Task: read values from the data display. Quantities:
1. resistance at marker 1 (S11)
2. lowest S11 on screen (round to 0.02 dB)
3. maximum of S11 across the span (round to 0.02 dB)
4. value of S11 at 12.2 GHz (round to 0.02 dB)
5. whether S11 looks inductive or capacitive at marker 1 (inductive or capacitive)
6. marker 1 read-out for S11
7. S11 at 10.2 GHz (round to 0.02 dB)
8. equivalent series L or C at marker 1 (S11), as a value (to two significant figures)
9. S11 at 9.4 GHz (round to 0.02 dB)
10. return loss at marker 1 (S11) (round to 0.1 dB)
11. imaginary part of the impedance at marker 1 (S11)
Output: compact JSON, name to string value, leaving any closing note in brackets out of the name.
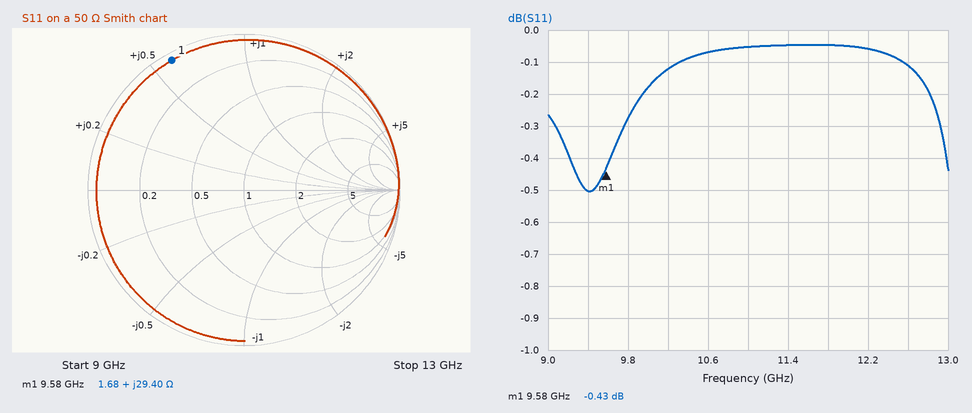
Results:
{"resistance at marker 1": "1.68 Ω", "lowest S11 on screen": "-0.50 dB", "maximum of S11 across the span": "-0.04 dB", "value of S11 at 12.2 GHz": "-0.06 dB", "whether S11 looks inductive or capacitive at marker 1": "inductive", "marker 1 read-out for S11": "-0.43 dB", "S11 at 10.2 GHz": "-0.12 dB", "equivalent series L or C at marker 1 (S11), as a value": "490 pH", "S11 at 9.4 GHz": "-0.50 dB", "return loss at marker 1 (S11)": "0.4 dB", "imaginary part of the impedance at marker 1": "+29.40 Ω"}
